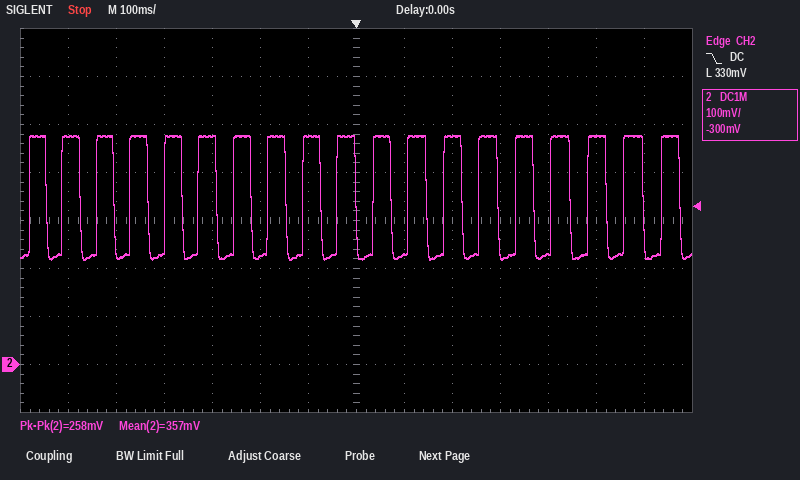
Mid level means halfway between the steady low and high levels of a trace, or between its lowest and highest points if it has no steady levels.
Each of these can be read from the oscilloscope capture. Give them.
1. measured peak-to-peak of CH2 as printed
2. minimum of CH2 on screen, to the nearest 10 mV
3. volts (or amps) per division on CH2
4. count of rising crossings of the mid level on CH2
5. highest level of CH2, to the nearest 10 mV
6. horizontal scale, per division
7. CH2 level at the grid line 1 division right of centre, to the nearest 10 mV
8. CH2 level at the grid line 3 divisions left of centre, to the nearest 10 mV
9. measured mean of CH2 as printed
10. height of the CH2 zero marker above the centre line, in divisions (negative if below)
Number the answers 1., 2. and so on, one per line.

1. 258 mV
2. 220 mV
3. 100 mV
4. 19
5. 480 mV
6. 100 ms
7. 230 mV
8. 480 mV
9. 357 mV
10. -3.0 div
